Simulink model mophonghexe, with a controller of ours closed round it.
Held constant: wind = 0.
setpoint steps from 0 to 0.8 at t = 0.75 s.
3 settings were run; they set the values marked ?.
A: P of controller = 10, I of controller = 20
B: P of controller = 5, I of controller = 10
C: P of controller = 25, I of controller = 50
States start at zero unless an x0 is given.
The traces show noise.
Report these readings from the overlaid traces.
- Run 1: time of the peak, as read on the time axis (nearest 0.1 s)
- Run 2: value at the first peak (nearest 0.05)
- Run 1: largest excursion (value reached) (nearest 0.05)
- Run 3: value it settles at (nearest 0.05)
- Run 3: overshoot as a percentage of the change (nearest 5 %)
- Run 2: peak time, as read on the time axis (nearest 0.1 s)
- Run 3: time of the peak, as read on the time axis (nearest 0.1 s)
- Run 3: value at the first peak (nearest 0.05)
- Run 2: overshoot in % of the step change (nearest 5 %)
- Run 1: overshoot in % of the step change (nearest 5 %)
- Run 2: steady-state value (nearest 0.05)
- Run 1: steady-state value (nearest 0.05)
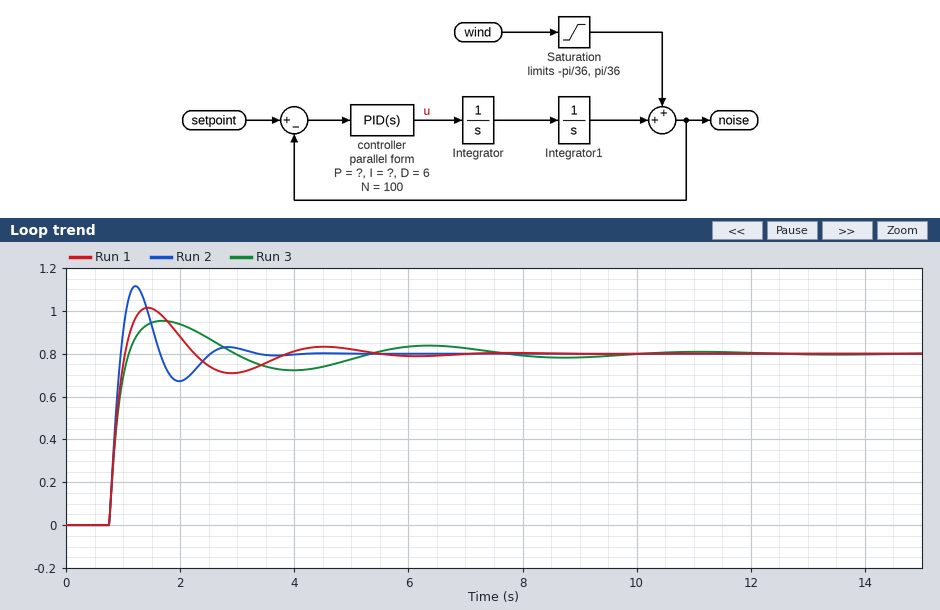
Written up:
1.4 s
1.10
1.00
0.80
20 %
1.2 s
1.7 s
0.95
40 %
25 %
0.80
0.80
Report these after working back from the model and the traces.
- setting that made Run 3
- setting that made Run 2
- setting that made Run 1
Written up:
B
C
A
